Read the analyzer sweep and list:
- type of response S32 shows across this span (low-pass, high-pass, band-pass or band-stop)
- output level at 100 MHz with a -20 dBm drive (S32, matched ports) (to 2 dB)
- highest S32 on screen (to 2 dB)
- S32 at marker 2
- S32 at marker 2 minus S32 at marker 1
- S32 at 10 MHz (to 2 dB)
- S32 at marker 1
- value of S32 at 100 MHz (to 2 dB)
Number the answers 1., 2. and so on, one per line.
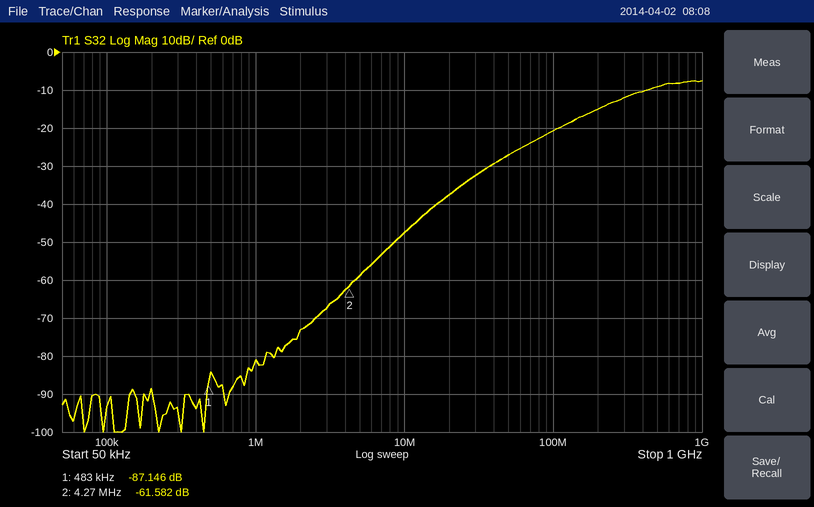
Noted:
1. high-pass
2. -40 dBm
3. -8 dB
4. -61.582 dB
5. 25.564 dB
6. -48 dB
7. -87.146 dB
8. -20 dB
